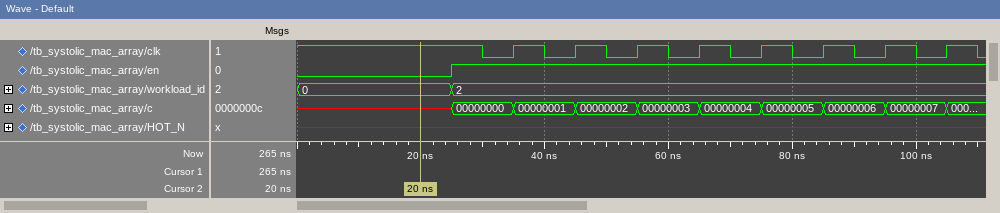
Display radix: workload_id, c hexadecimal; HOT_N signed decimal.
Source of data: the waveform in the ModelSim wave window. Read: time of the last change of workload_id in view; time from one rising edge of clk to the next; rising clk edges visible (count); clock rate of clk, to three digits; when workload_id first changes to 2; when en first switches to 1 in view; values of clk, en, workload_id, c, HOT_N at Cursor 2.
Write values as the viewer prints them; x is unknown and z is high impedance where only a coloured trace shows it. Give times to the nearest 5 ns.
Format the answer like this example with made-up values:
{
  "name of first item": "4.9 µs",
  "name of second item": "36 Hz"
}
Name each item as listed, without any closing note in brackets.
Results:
{
  "time of the last change of workload_id in view": "25 ns",
  "time from one rising edge of clk to the next": "10 ns",
  "rising clk edges visible": "8",
  "clock rate of clk, to three digits": "100 MHz",
  "when workload_id first changes to 2": "25 ns",
  "when en first switches to 1 in view": "25 ns",
  "values of clk, en, workload_id, c, HOT_N at Cursor 2": "clk=1, en=0, workload_id=0, c=x, HOT_N=x"
}
